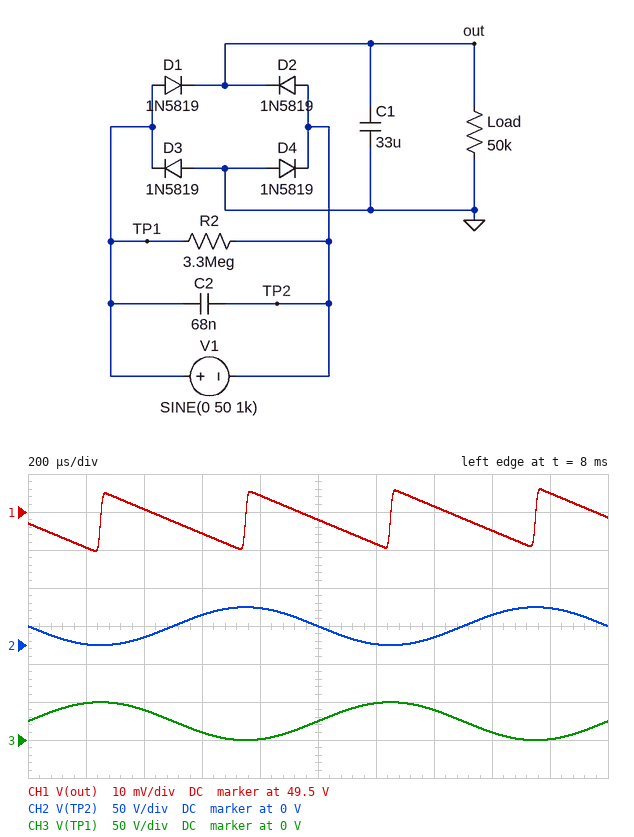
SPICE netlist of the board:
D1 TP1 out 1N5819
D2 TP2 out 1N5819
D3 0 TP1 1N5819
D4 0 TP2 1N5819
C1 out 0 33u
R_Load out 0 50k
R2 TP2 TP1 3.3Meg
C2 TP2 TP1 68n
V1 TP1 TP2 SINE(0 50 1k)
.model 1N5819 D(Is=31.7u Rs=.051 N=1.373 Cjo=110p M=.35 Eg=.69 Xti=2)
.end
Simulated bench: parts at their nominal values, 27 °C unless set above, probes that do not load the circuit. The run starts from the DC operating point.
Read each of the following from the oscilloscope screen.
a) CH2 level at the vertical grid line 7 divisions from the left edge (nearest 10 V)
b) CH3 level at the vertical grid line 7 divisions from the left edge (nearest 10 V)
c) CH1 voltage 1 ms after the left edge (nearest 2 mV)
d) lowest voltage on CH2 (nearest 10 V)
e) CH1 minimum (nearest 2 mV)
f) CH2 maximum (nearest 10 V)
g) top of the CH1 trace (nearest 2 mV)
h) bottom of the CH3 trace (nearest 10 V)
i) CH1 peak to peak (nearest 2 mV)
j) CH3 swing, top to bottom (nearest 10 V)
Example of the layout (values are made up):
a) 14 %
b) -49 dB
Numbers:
a) 10 V
b) 40 V
c) 49.498 V
d) 0 V
e) 49.490 V
f) 50 V
g) 49.506 V
h) 0 V
i) 16 mV
j) 50 V
